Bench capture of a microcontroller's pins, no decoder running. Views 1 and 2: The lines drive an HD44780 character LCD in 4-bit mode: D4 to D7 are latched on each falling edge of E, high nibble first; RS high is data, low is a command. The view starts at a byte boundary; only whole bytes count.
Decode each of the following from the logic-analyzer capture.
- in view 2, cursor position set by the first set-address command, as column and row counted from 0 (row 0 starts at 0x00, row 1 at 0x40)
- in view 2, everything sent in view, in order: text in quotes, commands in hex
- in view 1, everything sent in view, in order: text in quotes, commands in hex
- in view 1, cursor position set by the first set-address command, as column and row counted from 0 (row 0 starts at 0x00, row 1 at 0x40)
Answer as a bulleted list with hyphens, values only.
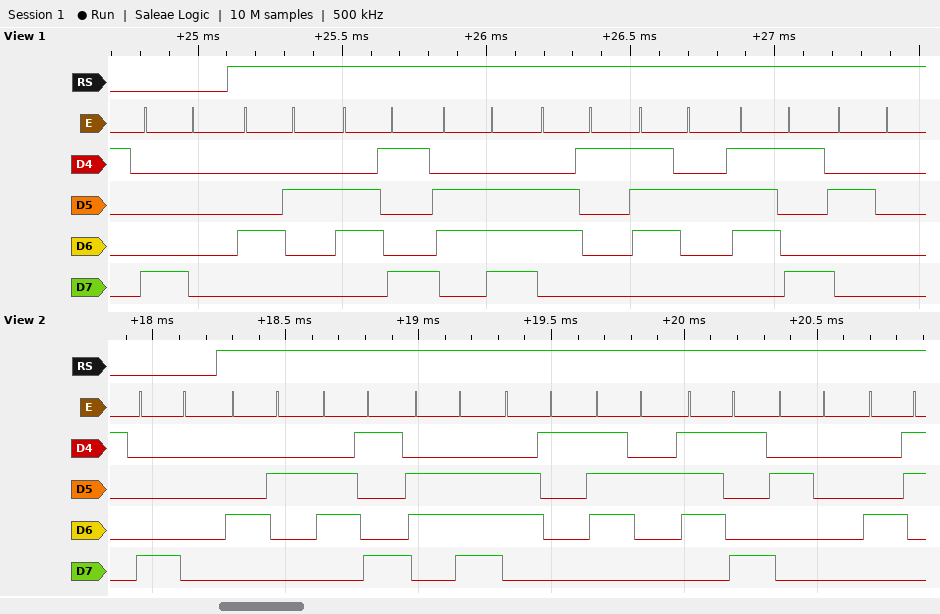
- column 0, row 0
- 0x80 "Binary C"
- 0x80 "Binary "
- column 0, row 0
